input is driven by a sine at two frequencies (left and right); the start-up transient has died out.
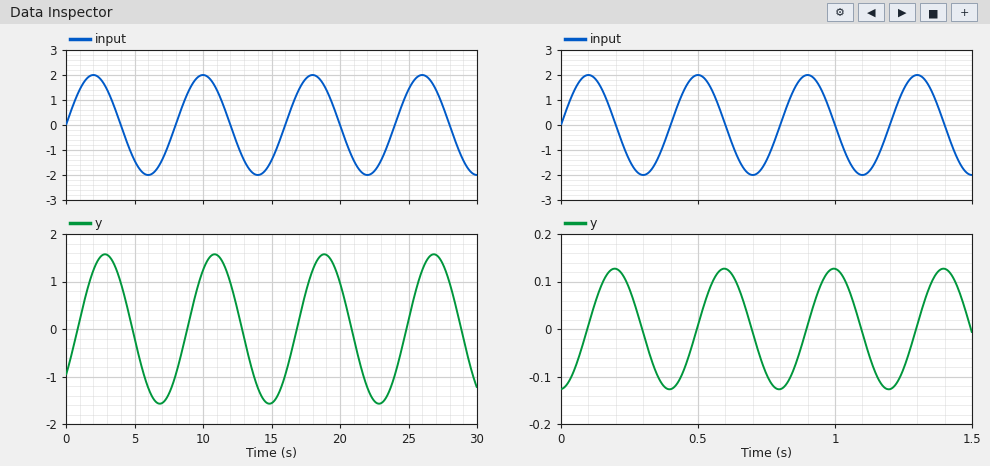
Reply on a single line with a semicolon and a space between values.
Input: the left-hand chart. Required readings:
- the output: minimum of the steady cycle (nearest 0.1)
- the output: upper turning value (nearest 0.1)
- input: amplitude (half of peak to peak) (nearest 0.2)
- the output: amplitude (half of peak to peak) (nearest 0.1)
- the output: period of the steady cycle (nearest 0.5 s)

-1.6; 1.6; 2.0; 1.6; 8.0 s
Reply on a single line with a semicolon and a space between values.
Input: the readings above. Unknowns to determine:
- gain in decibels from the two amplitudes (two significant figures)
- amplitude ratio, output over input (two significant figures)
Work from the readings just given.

-1.9 dB; 0.80
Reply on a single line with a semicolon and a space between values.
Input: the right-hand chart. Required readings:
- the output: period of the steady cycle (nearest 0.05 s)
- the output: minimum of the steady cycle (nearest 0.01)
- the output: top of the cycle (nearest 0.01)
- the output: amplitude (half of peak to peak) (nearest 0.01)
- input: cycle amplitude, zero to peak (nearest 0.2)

0.40 s; -0.13; 0.13; 0.13; 2.0
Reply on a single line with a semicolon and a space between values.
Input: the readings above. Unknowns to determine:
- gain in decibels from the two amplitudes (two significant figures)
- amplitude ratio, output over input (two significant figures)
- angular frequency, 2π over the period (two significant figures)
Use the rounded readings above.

-24 dB; 0.065; 16 rad/s
